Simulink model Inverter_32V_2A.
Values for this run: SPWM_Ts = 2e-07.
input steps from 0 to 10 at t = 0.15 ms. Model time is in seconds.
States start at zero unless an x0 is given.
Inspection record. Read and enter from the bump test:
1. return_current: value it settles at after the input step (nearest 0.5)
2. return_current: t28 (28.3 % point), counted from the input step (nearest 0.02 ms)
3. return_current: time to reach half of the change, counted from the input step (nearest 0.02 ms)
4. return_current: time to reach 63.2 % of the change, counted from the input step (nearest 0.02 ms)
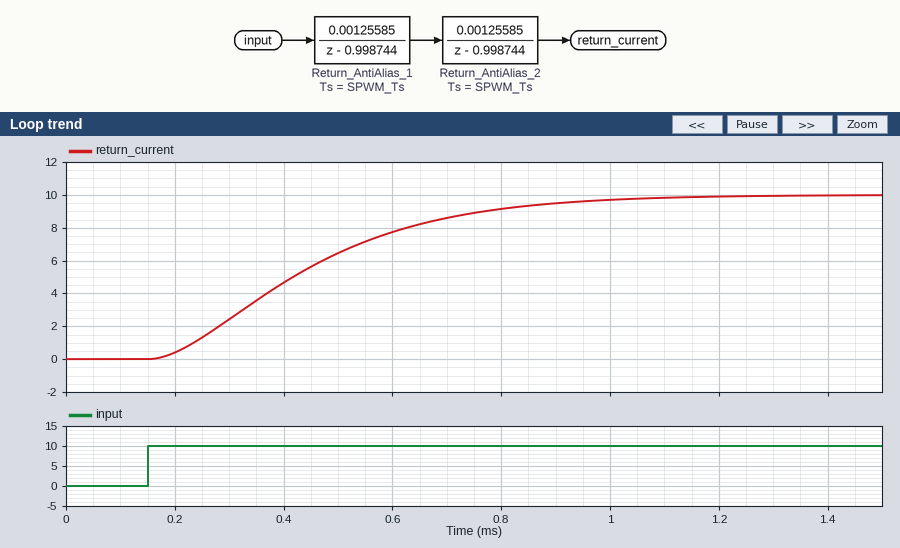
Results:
10.0
0.16 ms
0.26 ms
0.34 ms
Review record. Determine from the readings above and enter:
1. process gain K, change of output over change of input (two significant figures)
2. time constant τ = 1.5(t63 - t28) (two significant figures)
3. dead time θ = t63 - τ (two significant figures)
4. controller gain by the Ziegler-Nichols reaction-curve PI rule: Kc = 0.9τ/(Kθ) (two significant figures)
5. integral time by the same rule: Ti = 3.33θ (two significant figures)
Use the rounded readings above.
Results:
1.0
0.27 ms
0.070 ms
3.5
0.23 ms
